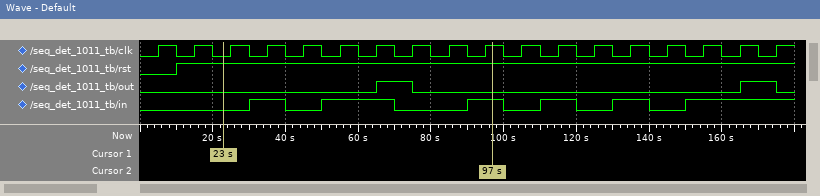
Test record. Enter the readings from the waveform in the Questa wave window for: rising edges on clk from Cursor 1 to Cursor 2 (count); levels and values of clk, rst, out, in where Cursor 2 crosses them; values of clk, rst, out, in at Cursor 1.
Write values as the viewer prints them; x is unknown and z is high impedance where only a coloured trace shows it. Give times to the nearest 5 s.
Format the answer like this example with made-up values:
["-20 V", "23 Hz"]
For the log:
["8", "clk=1, rst=1, out=0, in=1", "clk=0, rst=1, out=0, in=0"]
